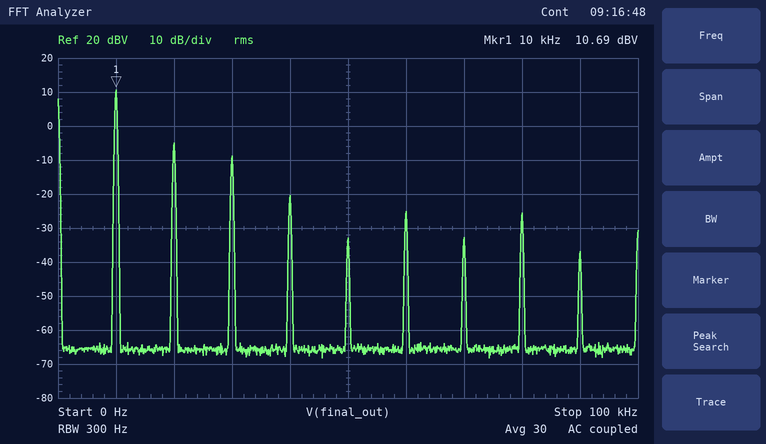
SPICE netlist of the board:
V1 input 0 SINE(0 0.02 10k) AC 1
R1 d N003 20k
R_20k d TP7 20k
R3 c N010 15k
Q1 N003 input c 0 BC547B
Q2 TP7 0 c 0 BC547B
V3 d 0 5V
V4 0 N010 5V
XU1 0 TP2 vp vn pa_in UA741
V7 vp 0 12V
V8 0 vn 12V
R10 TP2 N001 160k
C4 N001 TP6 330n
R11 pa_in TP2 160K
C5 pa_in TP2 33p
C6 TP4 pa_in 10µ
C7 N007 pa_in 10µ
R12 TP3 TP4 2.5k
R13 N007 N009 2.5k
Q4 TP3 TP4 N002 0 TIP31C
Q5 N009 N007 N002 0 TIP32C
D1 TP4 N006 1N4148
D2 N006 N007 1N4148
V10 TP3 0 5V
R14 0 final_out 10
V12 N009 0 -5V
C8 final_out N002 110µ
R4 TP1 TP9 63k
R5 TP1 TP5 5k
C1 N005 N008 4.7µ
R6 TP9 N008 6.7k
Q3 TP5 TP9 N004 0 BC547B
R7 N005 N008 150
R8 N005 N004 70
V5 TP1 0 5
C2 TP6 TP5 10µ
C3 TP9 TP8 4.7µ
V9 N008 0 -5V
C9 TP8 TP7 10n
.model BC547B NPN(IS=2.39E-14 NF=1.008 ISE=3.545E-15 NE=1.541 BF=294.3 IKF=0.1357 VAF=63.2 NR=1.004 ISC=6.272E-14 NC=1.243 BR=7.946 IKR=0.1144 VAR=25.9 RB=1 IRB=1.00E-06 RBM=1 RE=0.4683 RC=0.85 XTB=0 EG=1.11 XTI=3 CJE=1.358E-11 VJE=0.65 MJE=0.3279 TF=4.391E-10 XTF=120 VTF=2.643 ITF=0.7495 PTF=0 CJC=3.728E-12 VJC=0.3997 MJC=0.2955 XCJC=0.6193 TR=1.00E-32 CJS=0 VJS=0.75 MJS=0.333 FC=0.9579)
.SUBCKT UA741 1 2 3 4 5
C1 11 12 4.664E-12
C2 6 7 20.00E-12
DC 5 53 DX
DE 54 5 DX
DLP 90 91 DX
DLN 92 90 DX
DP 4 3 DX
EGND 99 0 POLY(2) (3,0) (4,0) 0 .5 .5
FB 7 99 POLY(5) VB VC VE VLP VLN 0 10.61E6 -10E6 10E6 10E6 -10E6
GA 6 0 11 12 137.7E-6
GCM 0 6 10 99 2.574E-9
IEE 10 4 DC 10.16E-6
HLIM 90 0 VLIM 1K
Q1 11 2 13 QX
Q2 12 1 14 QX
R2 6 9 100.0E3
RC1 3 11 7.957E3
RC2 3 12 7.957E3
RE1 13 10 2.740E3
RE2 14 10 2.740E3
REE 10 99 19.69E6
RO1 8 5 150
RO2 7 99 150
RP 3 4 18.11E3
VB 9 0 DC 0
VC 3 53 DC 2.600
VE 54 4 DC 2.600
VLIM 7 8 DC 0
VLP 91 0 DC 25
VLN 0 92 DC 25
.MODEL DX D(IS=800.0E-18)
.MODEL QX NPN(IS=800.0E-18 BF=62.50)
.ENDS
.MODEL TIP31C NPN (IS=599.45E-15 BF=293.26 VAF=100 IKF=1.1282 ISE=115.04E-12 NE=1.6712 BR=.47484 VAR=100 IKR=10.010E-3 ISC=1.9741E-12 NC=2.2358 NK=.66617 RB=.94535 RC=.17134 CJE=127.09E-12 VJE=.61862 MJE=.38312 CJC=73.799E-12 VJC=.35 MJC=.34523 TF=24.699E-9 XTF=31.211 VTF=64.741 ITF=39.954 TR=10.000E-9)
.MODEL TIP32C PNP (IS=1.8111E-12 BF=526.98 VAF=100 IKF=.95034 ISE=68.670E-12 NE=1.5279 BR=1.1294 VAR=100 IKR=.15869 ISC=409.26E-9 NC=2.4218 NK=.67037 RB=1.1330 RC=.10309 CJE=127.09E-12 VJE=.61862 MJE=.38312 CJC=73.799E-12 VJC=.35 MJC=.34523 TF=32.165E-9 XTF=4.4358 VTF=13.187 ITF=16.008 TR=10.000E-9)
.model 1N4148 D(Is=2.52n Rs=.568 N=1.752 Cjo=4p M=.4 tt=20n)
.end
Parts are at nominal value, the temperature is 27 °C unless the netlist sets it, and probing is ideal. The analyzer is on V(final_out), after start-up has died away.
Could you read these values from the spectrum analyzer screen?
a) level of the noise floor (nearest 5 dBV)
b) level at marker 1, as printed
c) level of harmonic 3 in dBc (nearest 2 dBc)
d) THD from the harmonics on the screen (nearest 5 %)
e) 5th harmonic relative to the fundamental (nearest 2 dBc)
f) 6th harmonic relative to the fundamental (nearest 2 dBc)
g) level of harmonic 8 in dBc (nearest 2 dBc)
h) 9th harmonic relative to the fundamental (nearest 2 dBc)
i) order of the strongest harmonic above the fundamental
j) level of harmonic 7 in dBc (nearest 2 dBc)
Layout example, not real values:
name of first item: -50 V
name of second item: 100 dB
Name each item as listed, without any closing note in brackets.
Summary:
level of the noise floor: -65 dBV
level at marker 1, as printed: 10.69 dBV
level of harmonic 3 in dBc: -20 dBc
THD from the harmonics on the screen: 20 %
5th harmonic relative to the fundamental: -44 dBc
6th harmonic relative to the fundamental: -36 dBc
level of harmonic 8 in dBc: -36 dBc
9th harmonic relative to the fundamental: -48 dBc
order of the strongest harmonic above the fundamental: 2
level of harmonic 7 in dBc: -44 dBc
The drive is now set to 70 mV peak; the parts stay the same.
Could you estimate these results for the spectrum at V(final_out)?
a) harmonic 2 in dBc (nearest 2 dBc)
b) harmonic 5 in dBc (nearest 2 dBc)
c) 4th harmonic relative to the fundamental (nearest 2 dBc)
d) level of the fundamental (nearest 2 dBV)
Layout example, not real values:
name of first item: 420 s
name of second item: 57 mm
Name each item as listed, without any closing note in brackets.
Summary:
harmonic 2 in dBc: -28 dBc
harmonic 5 in dBc: -38 dBc
4th harmonic relative to the fundamental: -40 dBc
level of the fundamental: 12 dBV
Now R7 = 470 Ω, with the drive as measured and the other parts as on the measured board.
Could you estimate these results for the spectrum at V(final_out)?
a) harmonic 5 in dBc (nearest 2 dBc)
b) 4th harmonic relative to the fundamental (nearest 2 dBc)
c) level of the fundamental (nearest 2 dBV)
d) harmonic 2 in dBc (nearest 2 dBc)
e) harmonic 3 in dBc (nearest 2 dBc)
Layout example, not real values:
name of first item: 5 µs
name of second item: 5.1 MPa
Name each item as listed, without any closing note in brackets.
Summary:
harmonic 5 in dBc: -38 dBc
4th harmonic relative to the fundamental: -26 dBc
level of the fundamental: 10 dBV
harmonic 2 in dBc: -12 dBc
harmonic 3 in dBc: -26 dBc
